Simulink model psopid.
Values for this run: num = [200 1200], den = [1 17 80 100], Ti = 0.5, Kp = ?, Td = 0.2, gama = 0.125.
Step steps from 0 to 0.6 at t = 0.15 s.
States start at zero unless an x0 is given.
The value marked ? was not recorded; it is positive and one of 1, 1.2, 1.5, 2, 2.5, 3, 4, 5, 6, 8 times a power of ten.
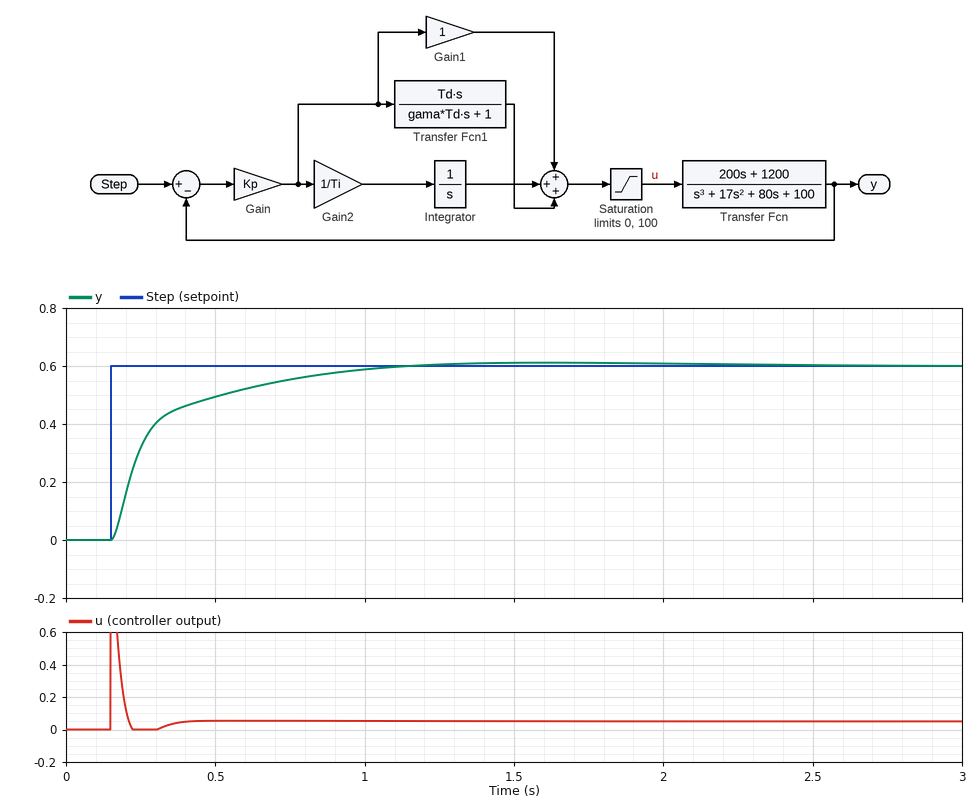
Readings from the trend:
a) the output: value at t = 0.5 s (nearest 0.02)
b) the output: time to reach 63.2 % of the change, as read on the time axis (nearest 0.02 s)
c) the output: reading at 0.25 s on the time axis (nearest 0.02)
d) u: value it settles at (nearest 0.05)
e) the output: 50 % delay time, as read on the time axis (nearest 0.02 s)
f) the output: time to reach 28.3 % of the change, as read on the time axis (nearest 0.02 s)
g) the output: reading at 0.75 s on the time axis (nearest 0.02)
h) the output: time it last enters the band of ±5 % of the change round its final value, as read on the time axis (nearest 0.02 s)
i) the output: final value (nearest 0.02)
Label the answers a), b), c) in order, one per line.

a) 0.50
b) 0.28 s
c) 0.32
d) 0.05
e) 0.24 s
f) 0.20 s
g) 0.56
h) 0.86 s
i) 0.60
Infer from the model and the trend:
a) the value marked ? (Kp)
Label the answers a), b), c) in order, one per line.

a) 0.25
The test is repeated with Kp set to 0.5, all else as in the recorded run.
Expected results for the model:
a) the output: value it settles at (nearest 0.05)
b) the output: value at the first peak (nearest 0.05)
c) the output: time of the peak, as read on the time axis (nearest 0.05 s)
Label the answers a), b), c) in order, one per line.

a) 0.60
b) 0.75
c) 0.40 s
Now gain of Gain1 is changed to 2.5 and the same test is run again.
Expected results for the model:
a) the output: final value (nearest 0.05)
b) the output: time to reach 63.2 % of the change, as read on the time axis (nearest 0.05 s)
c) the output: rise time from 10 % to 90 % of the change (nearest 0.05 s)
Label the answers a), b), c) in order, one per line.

a) 0.60
b) 0.25 s
c) 0.15 s
